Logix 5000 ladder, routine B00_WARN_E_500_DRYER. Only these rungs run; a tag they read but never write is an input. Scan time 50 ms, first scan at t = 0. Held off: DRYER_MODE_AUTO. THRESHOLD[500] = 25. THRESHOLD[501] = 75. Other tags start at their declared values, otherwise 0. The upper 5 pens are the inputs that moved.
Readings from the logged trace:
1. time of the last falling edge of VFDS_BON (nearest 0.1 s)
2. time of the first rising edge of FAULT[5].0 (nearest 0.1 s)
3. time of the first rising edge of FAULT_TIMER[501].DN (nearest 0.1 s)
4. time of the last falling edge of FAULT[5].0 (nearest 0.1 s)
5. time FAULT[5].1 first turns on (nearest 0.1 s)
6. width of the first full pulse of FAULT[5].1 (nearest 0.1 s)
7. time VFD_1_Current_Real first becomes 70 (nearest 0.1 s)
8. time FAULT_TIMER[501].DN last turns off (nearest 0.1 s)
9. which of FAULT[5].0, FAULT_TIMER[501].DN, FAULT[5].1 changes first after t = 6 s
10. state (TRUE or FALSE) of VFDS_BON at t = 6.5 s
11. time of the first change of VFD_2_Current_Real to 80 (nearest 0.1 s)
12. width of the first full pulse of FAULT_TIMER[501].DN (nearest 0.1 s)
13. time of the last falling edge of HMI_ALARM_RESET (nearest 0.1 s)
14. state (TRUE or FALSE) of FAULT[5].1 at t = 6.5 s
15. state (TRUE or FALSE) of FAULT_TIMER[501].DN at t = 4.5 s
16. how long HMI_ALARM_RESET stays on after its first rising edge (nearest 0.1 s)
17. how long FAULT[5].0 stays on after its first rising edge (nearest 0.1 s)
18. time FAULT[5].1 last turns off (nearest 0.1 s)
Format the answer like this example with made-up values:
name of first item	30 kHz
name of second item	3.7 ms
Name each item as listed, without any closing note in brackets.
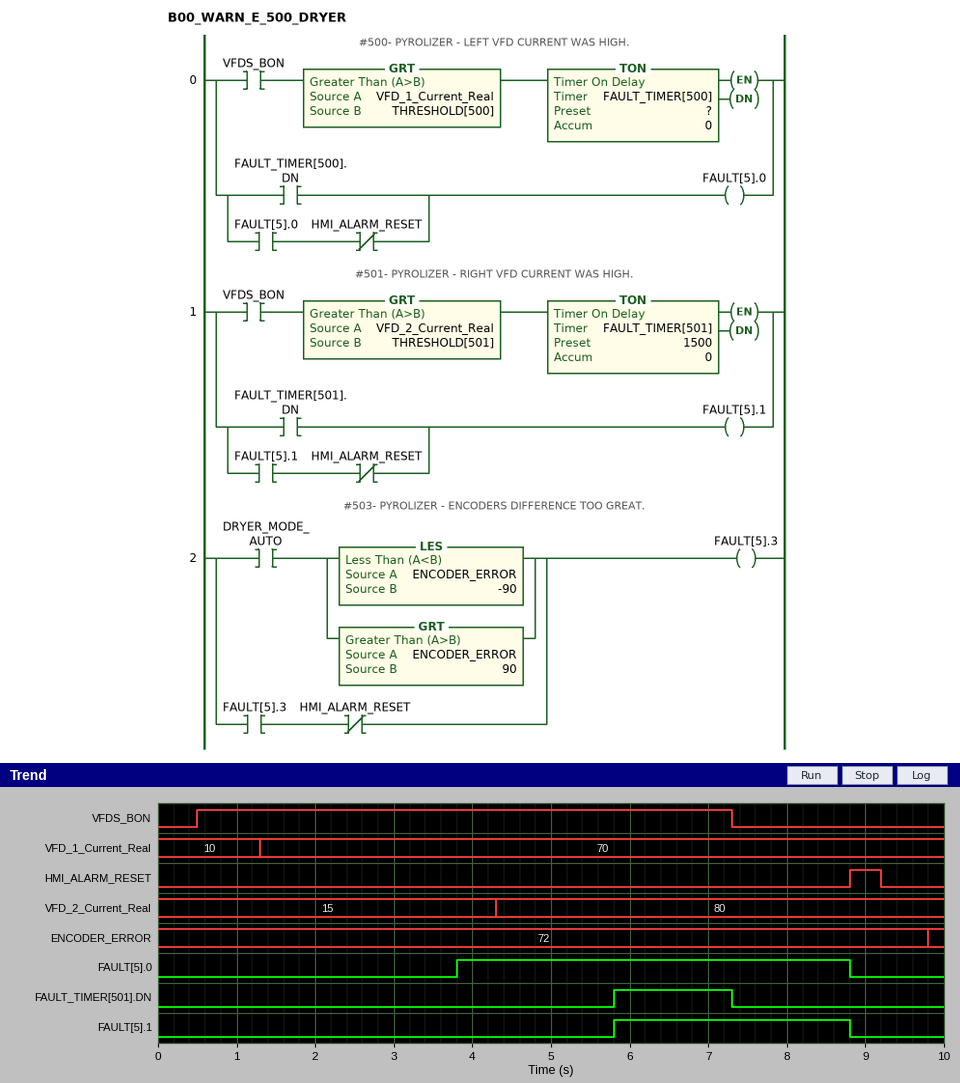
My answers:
time of the last falling edge of VFDS_BON	7.3 s
time of the first rising edge of FAULT[5].0	3.8 s
time of the first rising edge of FAULT_TIMER[501].DN	5.8 s
time of the last falling edge of FAULT[5].0	8.8 s
time FAULT[5].1 first turns on	5.8 s
width of the first full pulse of FAULT[5].1	3.0 s
time VFD_1_Current_Real first becomes 70	1.3 s
time FAULT_TIMER[501].DN last turns off	7.3 s
which of FAULT[5].0, FAULT_TIMER[501].DN, FAULT[5].1 changes first after t = 6 s	FAULT_TIMER[501].DN
state (TRUE or FALSE) of VFDS_BON at t = 6.5 s	TRUE
time of the first change of VFD_2_Current_Real to 80	4.3 s
width of the first full pulse of FAULT_TIMER[501].DN	1.5 s
time of the last falling edge of HMI_ALARM_RESET	9.2 s
state (TRUE or FALSE) of FAULT[5].1 at t = 6.5 s	TRUE
state (TRUE or FALSE) of FAULT_TIMER[501].DN at t = 4.5 s	FALSE
how long HMI_ALARM_RESET stays on after its first rising edge	0.4 s
how long FAULT[5].0 stays on after its first rising edge	5.0 s
time FAULT[5].1 last turns off	8.8 s
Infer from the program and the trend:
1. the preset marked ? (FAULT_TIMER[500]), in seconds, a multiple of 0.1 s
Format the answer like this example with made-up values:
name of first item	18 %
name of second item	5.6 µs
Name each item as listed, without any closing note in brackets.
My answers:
the preset marked ? (FAULT_TIMER[500]), in seconds, a multiple of 0.1 s	2.5 s
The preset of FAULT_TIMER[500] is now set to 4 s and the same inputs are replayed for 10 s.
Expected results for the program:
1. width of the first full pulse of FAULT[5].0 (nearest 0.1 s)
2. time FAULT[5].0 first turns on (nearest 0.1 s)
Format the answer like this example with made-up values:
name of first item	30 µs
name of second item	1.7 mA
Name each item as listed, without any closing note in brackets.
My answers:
width of the first full pulse of FAULT[5].0	3.5 s
time FAULT[5].0 first turns on	5.3 s
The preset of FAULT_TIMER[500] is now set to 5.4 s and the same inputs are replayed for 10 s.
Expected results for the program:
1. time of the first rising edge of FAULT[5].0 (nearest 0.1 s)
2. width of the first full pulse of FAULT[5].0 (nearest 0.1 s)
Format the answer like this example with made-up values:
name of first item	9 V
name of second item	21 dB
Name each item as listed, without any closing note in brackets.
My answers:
time of the first rising edge of FAULT[5].0	6.7 s
width of the first full pulse of FAULT[5].0	2.1 s
